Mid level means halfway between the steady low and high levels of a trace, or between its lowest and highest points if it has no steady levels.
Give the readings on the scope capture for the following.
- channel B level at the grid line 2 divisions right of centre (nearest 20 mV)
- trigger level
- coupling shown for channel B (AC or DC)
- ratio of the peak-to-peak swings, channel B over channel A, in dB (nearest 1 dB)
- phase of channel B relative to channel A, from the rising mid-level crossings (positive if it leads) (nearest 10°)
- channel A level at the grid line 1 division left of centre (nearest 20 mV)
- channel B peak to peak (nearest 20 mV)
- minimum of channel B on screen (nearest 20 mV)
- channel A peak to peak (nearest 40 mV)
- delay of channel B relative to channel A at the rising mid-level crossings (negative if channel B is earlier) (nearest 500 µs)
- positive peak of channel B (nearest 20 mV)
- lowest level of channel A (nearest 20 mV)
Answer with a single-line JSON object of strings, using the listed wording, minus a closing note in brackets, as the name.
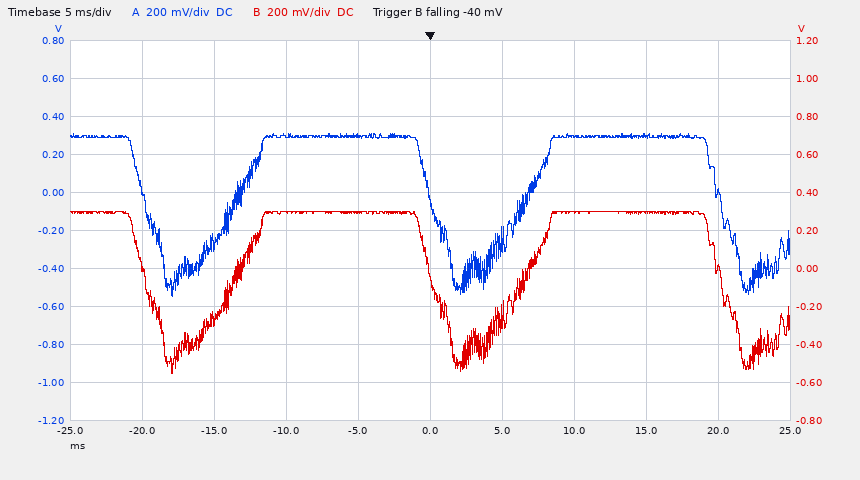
{"channel B level at the grid line 2 divisions right of centre": "300 mV", "trigger level": "-40 mV", "coupling shown for channel B": "DC", "ratio of the peak-to-peak swings, channel B over channel A, in dB": "0 dB", "phase of channel B relative to channel A, from the rising mid-level crossings (positive if it leads)": "0°", "channel A level at the grid line 1 division left of centre": "300 mV", "channel B peak to peak": "860 mV", "minimum of channel B on screen": "-560 mV", "channel A peak to peak": "840 mV", "delay of channel B relative to channel A at the rising mid-level crossings (negative if channel B is earlier)": "0.0 ms", "positive peak of channel B": "300 mV", "lowest level of channel A": "-540 mV"}
